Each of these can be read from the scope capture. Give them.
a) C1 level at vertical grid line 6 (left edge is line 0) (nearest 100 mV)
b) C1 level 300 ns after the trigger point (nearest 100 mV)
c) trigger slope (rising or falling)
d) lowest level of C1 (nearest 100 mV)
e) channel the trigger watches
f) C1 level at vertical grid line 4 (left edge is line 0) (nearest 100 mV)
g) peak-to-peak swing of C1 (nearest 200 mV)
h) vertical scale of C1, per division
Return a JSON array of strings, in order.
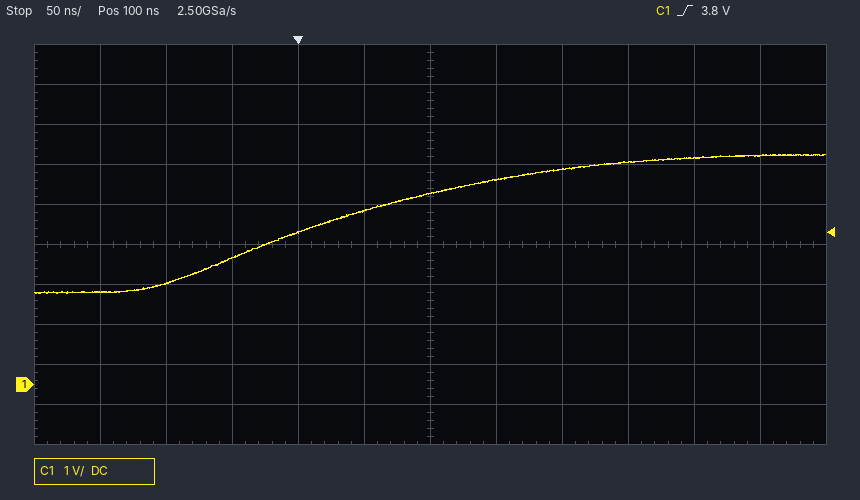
["4.8 V", "5.7 V", "rising", "2.3 V", "C1", "3.8 V", "3.4 V", "1 V"]
